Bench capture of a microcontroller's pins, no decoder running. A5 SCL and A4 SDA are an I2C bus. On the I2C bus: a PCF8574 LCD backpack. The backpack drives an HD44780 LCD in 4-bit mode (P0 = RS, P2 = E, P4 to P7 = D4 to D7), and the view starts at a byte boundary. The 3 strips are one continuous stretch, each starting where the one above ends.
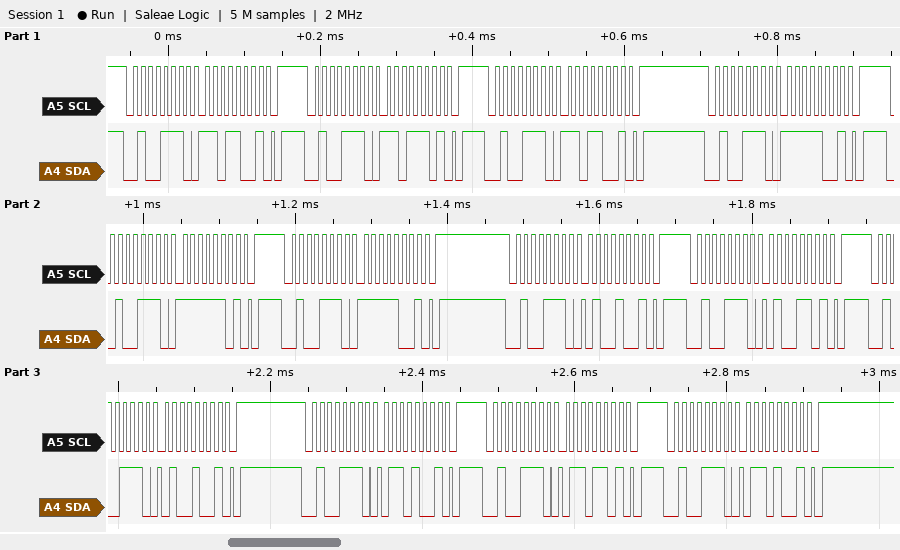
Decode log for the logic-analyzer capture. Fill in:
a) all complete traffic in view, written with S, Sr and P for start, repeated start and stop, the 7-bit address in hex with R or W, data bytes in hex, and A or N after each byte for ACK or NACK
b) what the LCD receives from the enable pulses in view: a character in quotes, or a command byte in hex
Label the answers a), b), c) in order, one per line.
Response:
a) S 27W A D9 A P S 27W A DD A P S 27W A D9 A P S 27W A F9 A P S 27W A FD A P S 27W A F9 A P S 27W A 49 A P S 27W A 4D A P S 27W A 49 A P S 27W A 69 A P S 27W A 6D A P S 27W A 69 A P
b) data 0xDF 'F'
